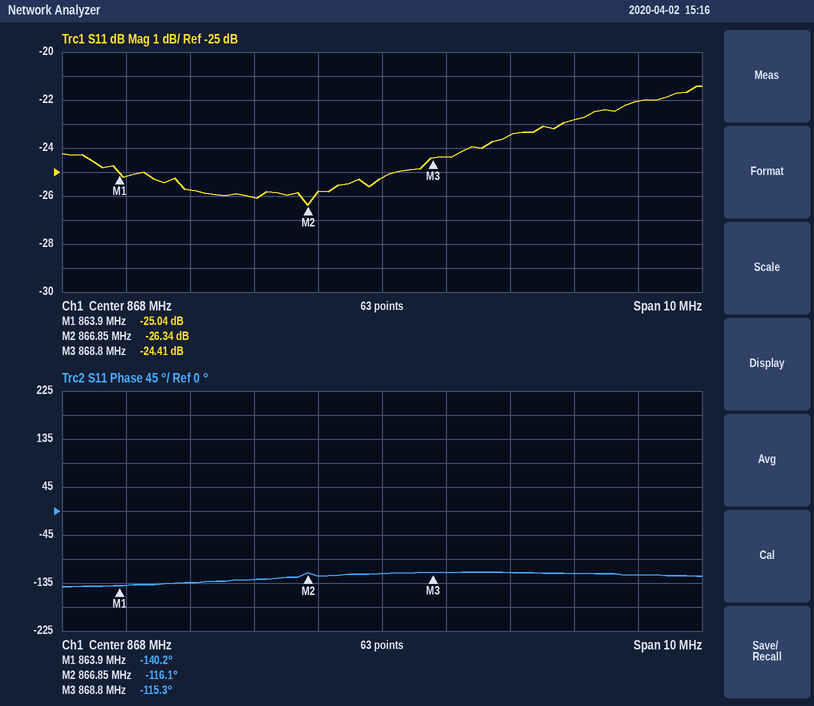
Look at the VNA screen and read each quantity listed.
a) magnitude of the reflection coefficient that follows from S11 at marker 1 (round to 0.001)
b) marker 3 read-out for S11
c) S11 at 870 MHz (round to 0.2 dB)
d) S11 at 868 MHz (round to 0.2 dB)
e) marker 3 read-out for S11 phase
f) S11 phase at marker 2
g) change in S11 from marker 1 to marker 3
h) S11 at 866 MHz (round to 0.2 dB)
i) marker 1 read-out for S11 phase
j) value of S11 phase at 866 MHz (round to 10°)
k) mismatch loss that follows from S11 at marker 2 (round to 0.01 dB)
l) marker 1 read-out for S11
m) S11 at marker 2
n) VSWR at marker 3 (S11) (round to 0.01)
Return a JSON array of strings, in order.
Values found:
["0.056", "-24.41 dB", "-23.4 dB", "-25.2 dB", "-115.3°", "-116.1°", "0.63 dB", "-26.0 dB", "-140.2°", "-130°", "0.01 dB", "-25.04 dB", "-26.34 dB", "1.13"]
